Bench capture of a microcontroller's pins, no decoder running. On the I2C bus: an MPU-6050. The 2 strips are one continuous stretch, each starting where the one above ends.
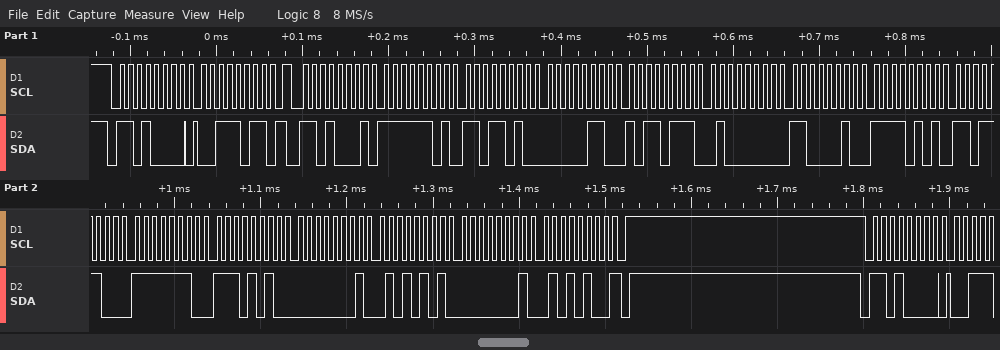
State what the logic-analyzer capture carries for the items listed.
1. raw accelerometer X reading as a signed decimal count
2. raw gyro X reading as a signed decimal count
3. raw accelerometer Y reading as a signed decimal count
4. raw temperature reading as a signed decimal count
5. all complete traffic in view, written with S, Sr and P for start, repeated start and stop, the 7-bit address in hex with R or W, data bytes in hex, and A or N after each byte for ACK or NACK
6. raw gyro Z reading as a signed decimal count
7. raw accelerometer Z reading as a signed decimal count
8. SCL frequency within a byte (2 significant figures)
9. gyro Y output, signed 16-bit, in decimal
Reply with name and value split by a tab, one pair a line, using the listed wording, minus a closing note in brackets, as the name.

raw accelerometer X reading as a signed decimal count	-550
raw gyro X reading as a signed decimal count	-278
raw accelerometer Y reading as a signed decimal count	1719
raw temperature reading as a signed decimal count	-2596
all complete traffic in view, written with S, Sr and P for start, repeated start and stop, the 7-bit address in hex with R or W, data bytes in hex, and A or N after each byte for ACK or NACK	S 68W A 3B A Sr 68R A FD A DA A 06 A B7 A 40 A C2 A F5 A DC A FE A EA A 01 A 55 A 01 A 54 N P S 68W A
raw gyro Z reading as a signed decimal count	340
raw accelerometer Z reading as a signed decimal count	16578
SCL frequency within a byte	100 kHz
gyro Y output, signed 16-bit, in decimal	341
